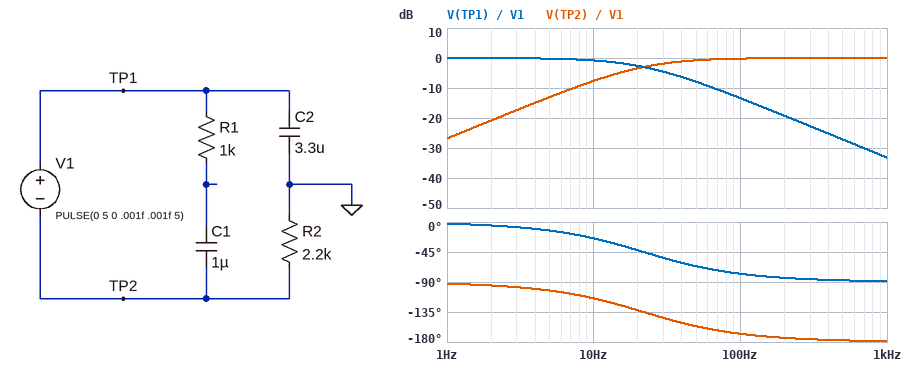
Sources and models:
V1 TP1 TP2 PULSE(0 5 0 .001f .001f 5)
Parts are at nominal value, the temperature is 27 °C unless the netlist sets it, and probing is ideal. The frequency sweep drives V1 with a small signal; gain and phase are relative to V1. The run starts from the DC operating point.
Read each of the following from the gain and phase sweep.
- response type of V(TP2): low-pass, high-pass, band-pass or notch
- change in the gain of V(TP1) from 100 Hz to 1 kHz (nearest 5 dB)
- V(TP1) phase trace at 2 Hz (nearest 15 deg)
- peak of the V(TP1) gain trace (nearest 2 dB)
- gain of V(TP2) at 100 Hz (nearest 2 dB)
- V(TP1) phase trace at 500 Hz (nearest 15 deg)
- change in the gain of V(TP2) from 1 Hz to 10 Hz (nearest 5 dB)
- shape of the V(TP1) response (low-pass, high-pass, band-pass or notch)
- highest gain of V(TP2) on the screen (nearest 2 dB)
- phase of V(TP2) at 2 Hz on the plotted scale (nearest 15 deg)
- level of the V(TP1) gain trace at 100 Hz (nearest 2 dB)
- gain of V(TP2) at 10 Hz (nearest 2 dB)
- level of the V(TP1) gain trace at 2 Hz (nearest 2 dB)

high-pass
-20 dB
0 deg
0 dB
0 dB
-90 deg
20 dB
low-pass
0 dB
-90 deg
-14 dB
-8 dB
0 dB
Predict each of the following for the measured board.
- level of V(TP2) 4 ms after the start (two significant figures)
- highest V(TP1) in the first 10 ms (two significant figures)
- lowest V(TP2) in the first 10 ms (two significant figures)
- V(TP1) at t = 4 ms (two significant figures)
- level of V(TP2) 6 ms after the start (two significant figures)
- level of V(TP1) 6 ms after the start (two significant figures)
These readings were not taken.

-2.9 V
3.7 V
-5.0 V
2.1 V
-2.2 V
2.8 V
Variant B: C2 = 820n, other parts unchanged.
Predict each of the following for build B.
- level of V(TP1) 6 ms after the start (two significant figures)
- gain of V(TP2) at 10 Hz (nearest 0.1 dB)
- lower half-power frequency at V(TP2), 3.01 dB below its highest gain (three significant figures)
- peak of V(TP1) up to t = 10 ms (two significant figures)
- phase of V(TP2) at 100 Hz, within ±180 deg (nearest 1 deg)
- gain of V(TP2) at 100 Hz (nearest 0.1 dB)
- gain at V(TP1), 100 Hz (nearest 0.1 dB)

4.8 V
-19.0 dB
88.2 Hz
5.0 V
-139 deg
-2.5 dB
-3.6 dB
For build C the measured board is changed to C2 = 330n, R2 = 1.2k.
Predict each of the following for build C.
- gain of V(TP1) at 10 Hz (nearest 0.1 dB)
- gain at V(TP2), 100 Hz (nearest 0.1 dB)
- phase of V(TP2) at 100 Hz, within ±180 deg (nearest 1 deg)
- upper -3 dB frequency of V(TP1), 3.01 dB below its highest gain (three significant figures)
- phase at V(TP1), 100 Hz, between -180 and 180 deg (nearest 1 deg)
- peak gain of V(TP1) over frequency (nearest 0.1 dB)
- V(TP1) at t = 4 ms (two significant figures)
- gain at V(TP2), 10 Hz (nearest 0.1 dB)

0 dB
-12.3 dB
-104 deg
402 Hz
-14 deg
0 dB
5.0 V
-32.1 dB
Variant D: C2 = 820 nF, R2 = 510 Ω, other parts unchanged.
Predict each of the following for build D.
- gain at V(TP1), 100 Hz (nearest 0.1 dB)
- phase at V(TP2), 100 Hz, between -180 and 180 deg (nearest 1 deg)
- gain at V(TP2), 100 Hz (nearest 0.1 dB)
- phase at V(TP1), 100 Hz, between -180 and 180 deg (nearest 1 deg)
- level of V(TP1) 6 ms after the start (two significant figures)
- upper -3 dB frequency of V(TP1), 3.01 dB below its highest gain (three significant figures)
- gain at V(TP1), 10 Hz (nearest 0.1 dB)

-0.3 dB
-105 deg
-11.9 dB
-15 deg
5.0 V
381 Hz
0 dB
